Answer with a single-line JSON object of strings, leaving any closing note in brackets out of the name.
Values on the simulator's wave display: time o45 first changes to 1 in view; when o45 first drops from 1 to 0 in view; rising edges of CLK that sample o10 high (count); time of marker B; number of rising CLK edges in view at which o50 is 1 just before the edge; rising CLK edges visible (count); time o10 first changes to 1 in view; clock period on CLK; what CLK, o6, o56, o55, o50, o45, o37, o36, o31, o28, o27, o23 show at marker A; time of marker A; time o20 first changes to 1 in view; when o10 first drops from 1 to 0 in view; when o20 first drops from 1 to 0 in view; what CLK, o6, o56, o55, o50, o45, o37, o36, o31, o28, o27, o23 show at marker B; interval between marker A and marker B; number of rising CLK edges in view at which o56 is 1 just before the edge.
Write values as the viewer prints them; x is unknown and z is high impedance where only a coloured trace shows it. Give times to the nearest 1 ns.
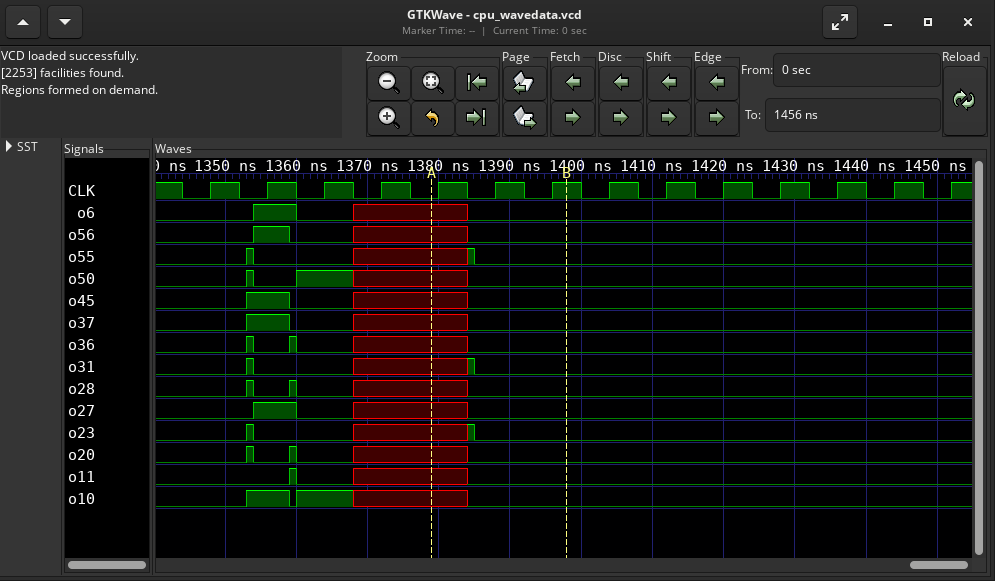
{"time o45 first changes to 1 in view": "1353 ns", "when o45 first drops from 1 to 0 in view": "1359 ns", "rising edges of CLK that sample o10 high": "2", "time of marker B": "1398 ns", "number of rising CLK edges in view at which o50 is 1 just before the edge": "1", "rising CLK edges visible": "14", "time o10 first changes to 1 in view": "1353 ns", "clock period on CLK": "8 ns", "what CLK, o6, o56, o55, o50, o45, o37, o36, o31, o28, o27, o23 show at marker A": "CLK=0, o6=x, o56=x, o55=x, o50=x, o45=x, o37=x, o36=x, o31=x, o28=x, o27=x, o23=x", "time of marker A": "1379 ns", "time o20 first changes to 1 in view": "1353 ns", "when o10 first drops from 1 to 0 in view": "1359 ns", "when o20 first drops from 1 to 0 in view": "1354 ns", "what CLK, o6, o56, o55, o50, o45, o37, o36, o31, o28, o27, o23 show at marker B": "CLK=1, o6=0, o56=0, o55=0, o50=0, o45=0, o37=0, o36=0, o31=0, o28=0, o27=0, o23=0", "interval between marker A and marker B": "19 ns", "number of rising CLK edges in view at which o56 is 1 just before the edge": "1"}
